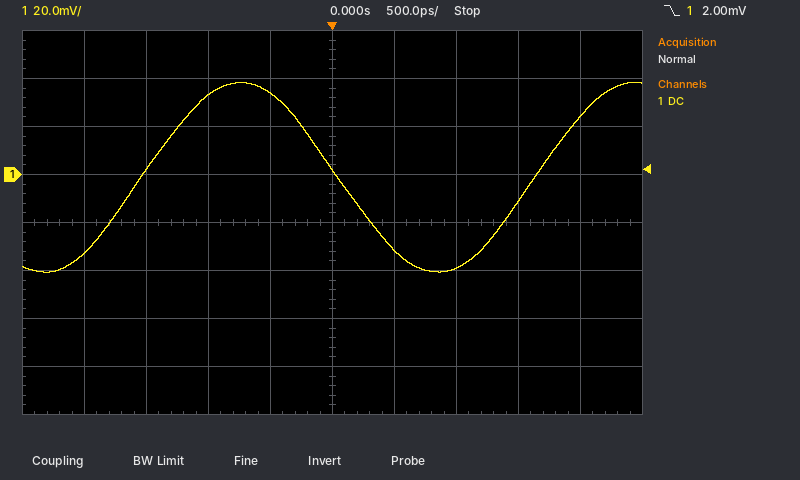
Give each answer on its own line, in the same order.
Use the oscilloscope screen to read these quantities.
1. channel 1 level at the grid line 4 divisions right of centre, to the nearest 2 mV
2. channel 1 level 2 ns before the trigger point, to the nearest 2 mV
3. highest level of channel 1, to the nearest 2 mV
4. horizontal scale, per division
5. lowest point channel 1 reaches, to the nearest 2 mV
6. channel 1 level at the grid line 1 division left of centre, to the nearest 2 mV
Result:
24 mV
-32 mV
38 mV
500 ps
-40 mV
34 mV
